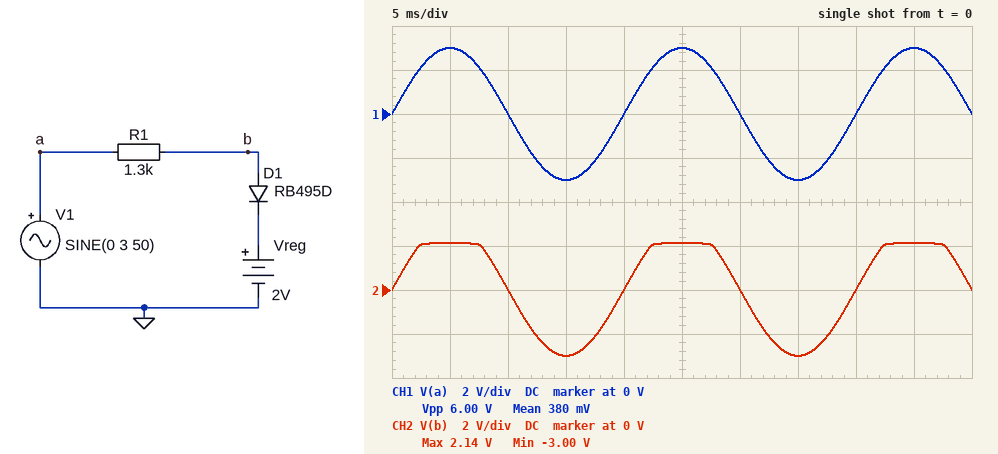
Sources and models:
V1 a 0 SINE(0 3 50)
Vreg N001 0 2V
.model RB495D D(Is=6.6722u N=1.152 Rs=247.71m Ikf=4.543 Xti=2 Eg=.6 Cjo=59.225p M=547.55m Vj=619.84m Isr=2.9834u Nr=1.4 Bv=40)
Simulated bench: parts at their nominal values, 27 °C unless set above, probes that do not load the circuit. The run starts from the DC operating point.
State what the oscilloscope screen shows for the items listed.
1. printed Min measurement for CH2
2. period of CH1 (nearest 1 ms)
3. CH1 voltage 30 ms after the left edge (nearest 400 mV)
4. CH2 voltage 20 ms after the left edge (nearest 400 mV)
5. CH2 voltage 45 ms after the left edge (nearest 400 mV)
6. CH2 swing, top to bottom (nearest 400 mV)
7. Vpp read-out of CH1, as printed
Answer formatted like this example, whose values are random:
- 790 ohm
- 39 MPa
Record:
- -3.00 V
- 20 ms
- 0 V
- 0 V
- 2.0 V
- 5.2 V
- 6.00 V
